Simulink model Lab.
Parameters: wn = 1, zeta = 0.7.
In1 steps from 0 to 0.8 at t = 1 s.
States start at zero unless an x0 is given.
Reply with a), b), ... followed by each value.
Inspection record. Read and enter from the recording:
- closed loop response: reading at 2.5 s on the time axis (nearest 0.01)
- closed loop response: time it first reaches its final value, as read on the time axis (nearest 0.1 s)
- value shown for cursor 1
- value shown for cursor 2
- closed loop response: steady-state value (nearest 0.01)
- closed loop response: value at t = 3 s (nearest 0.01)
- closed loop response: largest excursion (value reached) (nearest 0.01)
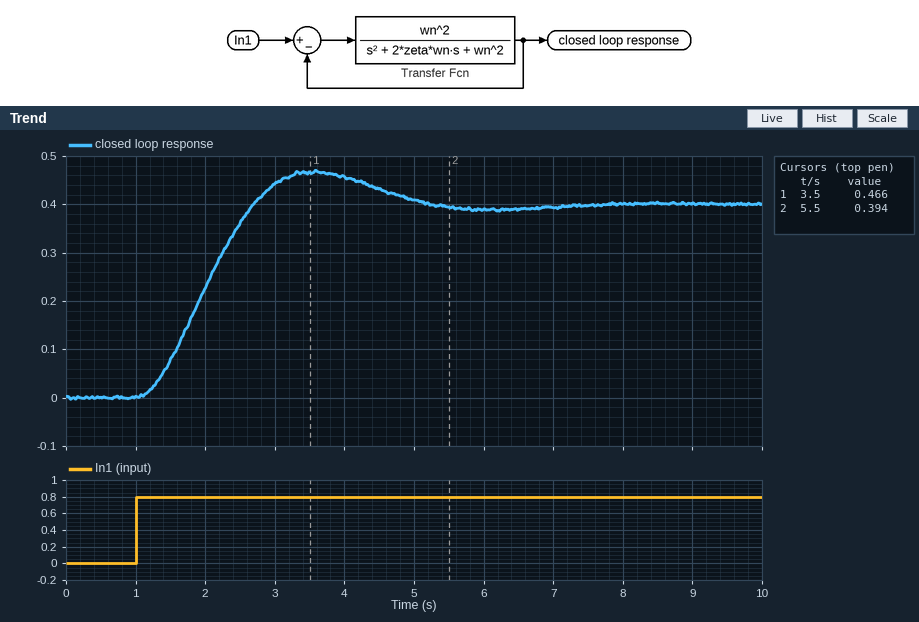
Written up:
a) 0.36
b) 2.7 s
c) 0.466
d) 0.394
e) 0.40
f) 0.44
g) 0.47
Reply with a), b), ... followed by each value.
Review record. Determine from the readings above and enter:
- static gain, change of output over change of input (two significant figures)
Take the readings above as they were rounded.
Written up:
a) 0.50
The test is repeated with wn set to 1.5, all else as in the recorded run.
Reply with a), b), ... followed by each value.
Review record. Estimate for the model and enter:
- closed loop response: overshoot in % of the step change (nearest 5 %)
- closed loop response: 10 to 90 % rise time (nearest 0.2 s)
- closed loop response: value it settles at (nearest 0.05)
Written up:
a) 15 %
b) 0.8 s
c) 0.40
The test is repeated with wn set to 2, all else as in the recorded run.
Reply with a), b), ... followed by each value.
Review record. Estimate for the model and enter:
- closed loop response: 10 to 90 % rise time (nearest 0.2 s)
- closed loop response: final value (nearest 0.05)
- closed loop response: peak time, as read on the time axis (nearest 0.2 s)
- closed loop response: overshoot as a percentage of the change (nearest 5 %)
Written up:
a) 0.6 s
b) 0.40
c) 2.2 s
d) 15 %
